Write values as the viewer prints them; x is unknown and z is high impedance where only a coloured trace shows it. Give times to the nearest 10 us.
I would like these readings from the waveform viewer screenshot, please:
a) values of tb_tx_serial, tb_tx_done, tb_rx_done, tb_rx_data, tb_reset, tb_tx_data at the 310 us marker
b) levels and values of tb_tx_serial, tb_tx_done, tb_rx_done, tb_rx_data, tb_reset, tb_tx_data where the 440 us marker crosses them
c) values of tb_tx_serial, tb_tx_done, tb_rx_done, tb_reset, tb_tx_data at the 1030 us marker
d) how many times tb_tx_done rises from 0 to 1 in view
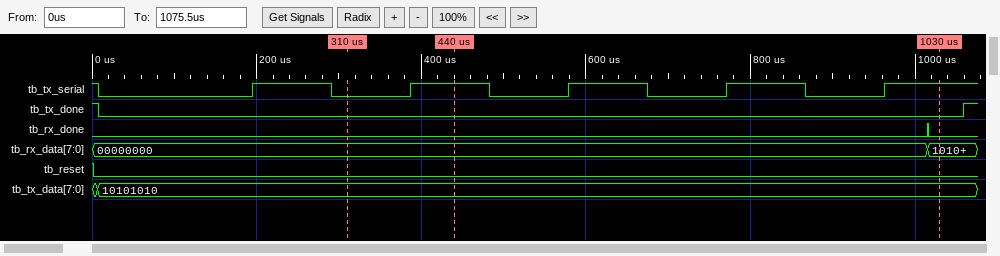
tb_tx_serial=0, tb_tx_done=0, tb_rx_done=0, tb_rx_data=00000000, tb_reset=0, tb_tx_data=10101010
tb_tx_serial=1, tb_tx_done=0, tb_rx_done=0, tb_rx_data=00000000, tb_reset=0, tb_tx_data=10101010
tb_tx_serial=1, tb_tx_done=0, tb_rx_done=0, tb_reset=0, tb_tx_data=10101010
1
